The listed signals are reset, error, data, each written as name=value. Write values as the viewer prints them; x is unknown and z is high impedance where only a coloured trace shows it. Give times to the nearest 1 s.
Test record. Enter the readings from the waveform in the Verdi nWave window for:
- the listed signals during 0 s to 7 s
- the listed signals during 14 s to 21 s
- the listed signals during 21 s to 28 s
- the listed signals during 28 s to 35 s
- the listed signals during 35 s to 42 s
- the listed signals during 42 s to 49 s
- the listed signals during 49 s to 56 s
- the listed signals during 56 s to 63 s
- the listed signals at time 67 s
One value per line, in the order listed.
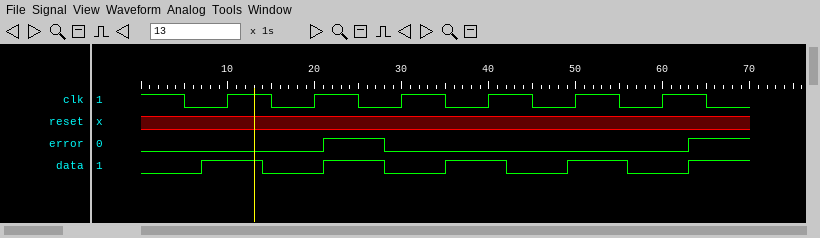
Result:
reset=x, error=0, data=0
reset=x, error=0, data=0
reset=x, error=1, data=1
reset=x, error=0, data=0
reset=x, error=0, data=1
reset=x, error=0, data=0
reset=x, error=0, data=1
reset=x, error=0, data=0
reset=x, error=1, data=1
